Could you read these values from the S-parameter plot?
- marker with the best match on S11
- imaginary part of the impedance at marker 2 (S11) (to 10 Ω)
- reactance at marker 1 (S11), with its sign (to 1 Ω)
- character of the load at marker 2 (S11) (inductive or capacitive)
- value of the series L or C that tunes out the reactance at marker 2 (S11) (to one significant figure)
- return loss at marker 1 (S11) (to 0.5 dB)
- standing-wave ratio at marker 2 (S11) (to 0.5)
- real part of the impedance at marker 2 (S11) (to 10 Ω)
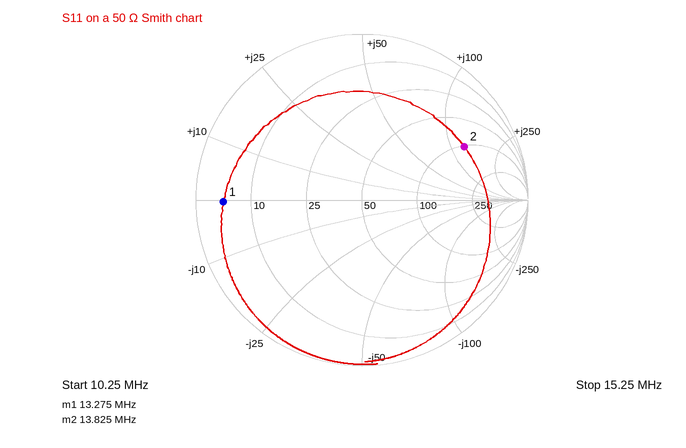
marker 2
+130 Ω
0 Ω
inductive
90 pF
1.5 dB
5.5
100 Ω
